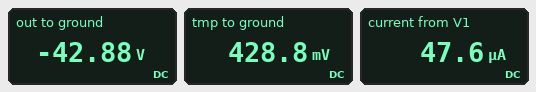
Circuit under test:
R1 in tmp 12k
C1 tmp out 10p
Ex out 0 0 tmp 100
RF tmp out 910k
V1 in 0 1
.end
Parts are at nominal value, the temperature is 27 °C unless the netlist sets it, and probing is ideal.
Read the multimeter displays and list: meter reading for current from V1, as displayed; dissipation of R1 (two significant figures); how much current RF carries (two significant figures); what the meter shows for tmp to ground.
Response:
47.6 µA
27 µW
48 µA
428.8 mV
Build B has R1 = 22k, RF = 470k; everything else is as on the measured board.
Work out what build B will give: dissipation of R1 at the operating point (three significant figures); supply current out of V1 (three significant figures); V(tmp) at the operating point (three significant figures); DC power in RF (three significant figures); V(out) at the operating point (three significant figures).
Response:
31.0 µW
37.5 µA
175 mV
662 µW
-17.5 V
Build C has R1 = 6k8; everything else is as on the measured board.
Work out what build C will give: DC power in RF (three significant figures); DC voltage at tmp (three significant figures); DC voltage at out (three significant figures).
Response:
3.64 mW
570 mV
-57.0 V
